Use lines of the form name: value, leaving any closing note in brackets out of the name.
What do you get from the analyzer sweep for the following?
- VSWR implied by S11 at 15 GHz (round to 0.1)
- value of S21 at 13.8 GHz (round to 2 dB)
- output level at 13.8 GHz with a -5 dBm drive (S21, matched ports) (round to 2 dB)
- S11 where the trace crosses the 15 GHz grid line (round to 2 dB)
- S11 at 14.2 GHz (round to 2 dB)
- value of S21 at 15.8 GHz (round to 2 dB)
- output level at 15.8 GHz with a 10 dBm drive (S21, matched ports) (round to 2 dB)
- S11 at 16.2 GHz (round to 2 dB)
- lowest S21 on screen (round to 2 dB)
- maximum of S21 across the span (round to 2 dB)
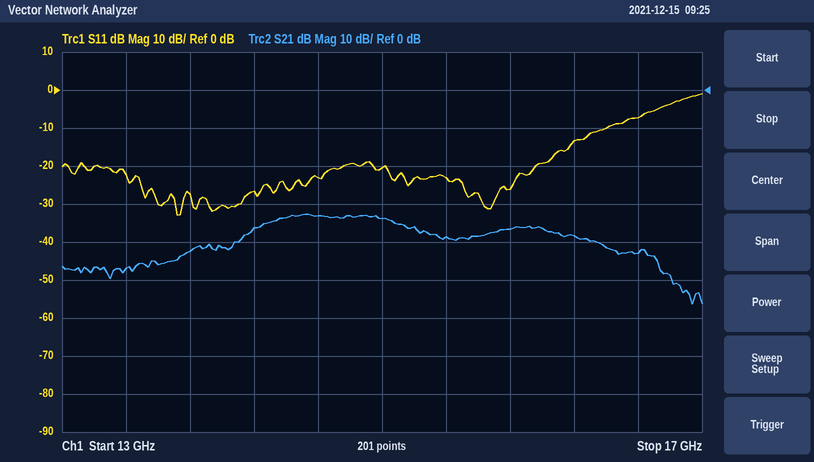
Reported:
VSWR implied by S11 at 15 GHz: 1.2
value of S21 at 13.8 GHz: -42 dB
output level at 13.8 GHz with a -5 dBm drive (S21, matched ports): -48 dBm
S11 where the trace crosses the 15 GHz grid line: -20 dB
S11 at 14.2 GHz: -26 dB
value of S21 at 15.8 GHz: -36 dB
output level at 15.8 GHz with a 10 dBm drive (S21, matched ports): -26 dBm
S11 at 16.2 GHz: -14 dB
lowest S21 on screen: -56 dB
maximum of S21 across the span: -32 dB
